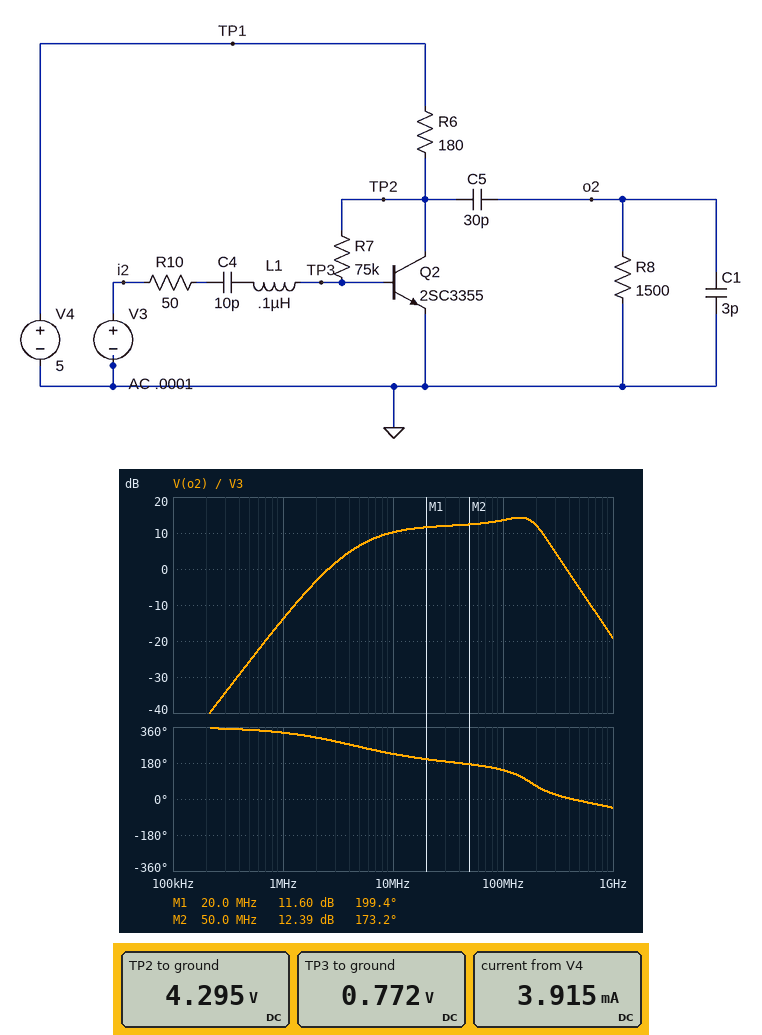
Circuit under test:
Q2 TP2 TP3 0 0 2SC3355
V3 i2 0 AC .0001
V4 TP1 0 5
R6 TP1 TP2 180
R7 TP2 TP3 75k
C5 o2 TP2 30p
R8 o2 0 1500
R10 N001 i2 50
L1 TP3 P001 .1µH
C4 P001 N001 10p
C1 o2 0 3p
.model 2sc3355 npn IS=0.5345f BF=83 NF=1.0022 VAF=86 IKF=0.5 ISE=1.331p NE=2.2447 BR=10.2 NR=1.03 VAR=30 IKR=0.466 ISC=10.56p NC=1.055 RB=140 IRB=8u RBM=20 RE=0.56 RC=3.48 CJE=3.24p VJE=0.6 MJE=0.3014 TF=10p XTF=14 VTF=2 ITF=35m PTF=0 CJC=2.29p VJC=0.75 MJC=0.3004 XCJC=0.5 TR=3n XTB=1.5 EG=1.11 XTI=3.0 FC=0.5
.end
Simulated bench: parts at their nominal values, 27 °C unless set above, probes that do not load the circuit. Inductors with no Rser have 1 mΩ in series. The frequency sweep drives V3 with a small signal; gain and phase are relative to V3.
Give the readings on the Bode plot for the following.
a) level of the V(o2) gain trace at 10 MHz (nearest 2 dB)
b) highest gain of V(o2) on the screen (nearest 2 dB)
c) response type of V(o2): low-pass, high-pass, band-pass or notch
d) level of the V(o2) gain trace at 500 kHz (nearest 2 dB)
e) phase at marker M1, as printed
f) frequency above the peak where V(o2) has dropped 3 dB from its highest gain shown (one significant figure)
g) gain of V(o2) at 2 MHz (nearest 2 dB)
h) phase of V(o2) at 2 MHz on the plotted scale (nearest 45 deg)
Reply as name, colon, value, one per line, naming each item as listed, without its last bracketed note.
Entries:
level of the V(o2) gain trace at 10 MHz: 10 dB
highest gain of V(o2) on the screen: 14 dB
response type of V(o2): low-pass, high-pass, band-pass or notch: band-pass
level of the V(o2) gain trace at 500 kHz: -26 dB
phase at marker M1, as printed: 199.4 deg
frequency above the peak where V(o2) has dropped 3 dB from its highest gain shown: 200 MHz
gain of V(o2) at 2 MHz: -4 dB
phase of V(o2) at 2 MHz on the plotted scale: 315 deg
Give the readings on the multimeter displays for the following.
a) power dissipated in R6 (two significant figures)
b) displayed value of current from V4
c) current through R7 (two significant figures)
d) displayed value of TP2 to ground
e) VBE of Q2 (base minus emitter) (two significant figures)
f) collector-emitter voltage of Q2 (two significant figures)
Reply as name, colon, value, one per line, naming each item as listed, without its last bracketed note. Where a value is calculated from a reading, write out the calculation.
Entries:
power dissipated in R6: (5 V - 4.295 V)^2 / 180 Ω = 2.8 mW
displayed value of current from V4: 3.915 mA
current through R7: (4.295 V - 772 mV) / 75 kΩ = 47 µA
displayed value of TP2 to ground: 4.295 V
VBE of Q2 (base minus emitter): 772 mV = 770 mV
collector-emitter voltage of Q2: 4.295 V = 4.3 V
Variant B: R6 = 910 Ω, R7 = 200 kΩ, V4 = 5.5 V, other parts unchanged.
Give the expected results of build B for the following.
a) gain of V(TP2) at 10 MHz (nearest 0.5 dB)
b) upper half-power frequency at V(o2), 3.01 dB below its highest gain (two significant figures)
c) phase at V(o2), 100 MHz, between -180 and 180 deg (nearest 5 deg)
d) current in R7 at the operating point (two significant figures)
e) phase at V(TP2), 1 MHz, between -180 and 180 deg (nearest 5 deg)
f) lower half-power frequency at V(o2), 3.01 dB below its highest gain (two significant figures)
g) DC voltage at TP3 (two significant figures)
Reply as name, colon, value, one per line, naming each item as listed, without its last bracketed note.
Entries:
gain of V(TP2) at 10 MHz: 14.0 dB
upper half-power frequency at V(o2), 3.01 dB below its highest gain: 190 MHz
phase at V(o2), 100 MHz, between -180 and 180 deg: 125 deg
current in R7 at the operating point: 17 µA
phase at V(TP2), 1 MHz, between -180 and 180 deg: -125 deg
lower half-power frequency at V(o2), 3.01 dB below its highest gain: 4.2 MHz
DC voltage at TP3: 740 mV
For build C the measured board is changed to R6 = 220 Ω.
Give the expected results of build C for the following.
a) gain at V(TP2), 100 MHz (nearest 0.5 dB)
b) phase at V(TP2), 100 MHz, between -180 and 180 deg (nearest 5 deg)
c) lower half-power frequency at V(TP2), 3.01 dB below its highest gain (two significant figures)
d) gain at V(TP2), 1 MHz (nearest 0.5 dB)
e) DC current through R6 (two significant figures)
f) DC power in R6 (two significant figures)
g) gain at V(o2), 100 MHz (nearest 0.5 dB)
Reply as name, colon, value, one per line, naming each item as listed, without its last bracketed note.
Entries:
gain at V(TP2), 100 MHz: 15.0 dB
phase at V(TP2), 100 MHz, between -180 and 180 deg: 140 deg
lower half-power frequency at V(TP2), 3.01 dB below its highest gain: 12 MHz
gain at V(TP2), 1 MHz: -1.0 dB
DC current through R6: 3.8 mA
DC power in R6: 3.1 mW
gain at V(o2), 100 MHz: 14.0 dB
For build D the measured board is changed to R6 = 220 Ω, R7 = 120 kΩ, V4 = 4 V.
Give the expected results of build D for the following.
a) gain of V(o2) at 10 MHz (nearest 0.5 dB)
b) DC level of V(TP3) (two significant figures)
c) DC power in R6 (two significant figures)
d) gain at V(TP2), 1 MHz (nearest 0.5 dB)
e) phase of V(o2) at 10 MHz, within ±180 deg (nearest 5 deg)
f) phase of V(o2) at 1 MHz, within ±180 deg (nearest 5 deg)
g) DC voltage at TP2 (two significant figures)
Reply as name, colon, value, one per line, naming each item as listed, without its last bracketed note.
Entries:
gain of V(o2) at 10 MHz: 9.0 dB
DC level of V(TP3): 750 mV
DC power in R6: 830 µW
gain at V(TP2), 1 MHz: -0.5 dB
phase of V(o2) at 10 MHz, within ±180 deg: -145 deg
phase of V(o2) at 1 MHz, within ±180 deg: -35 deg
DC voltage at TP2: 3.6 V
